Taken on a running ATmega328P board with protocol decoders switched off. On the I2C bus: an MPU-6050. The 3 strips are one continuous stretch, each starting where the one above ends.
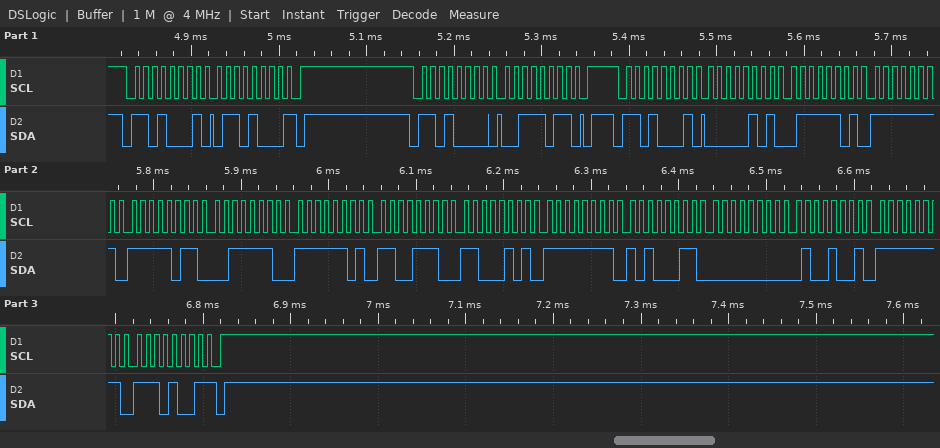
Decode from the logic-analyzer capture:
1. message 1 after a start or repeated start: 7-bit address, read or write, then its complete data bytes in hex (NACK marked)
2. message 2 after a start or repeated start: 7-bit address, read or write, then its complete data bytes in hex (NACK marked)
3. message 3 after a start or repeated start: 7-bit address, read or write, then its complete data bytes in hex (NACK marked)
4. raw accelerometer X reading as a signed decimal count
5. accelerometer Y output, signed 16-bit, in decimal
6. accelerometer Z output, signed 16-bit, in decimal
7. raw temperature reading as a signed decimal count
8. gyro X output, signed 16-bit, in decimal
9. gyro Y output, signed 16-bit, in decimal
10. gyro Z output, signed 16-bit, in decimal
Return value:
0x68 read: 68 NACK
0x68 write: 3B
0x68 read: 05 7D FF FB 3E FD CE C5 FF A3 00 49 FF E9 NACK
1405
-5
16125
-12603
-93
73
-23
